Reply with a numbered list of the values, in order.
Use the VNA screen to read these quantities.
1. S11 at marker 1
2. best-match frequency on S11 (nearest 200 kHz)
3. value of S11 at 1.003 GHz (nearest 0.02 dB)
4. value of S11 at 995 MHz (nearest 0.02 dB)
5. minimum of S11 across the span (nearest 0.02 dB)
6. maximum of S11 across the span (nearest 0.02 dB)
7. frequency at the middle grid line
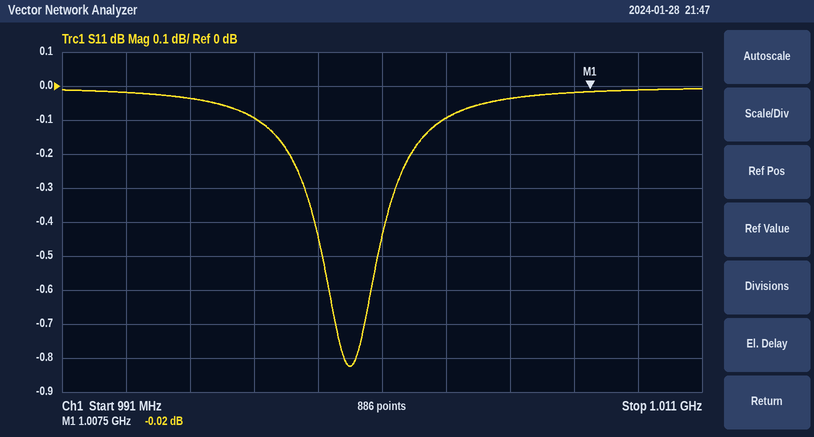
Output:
1. -0.02 dB
2. 1.0000 GHz
3. -0.10 dB
4. -0.04 dB
5. -0.82 dB
6. 0.00 dB
7. 1.001 GHz
